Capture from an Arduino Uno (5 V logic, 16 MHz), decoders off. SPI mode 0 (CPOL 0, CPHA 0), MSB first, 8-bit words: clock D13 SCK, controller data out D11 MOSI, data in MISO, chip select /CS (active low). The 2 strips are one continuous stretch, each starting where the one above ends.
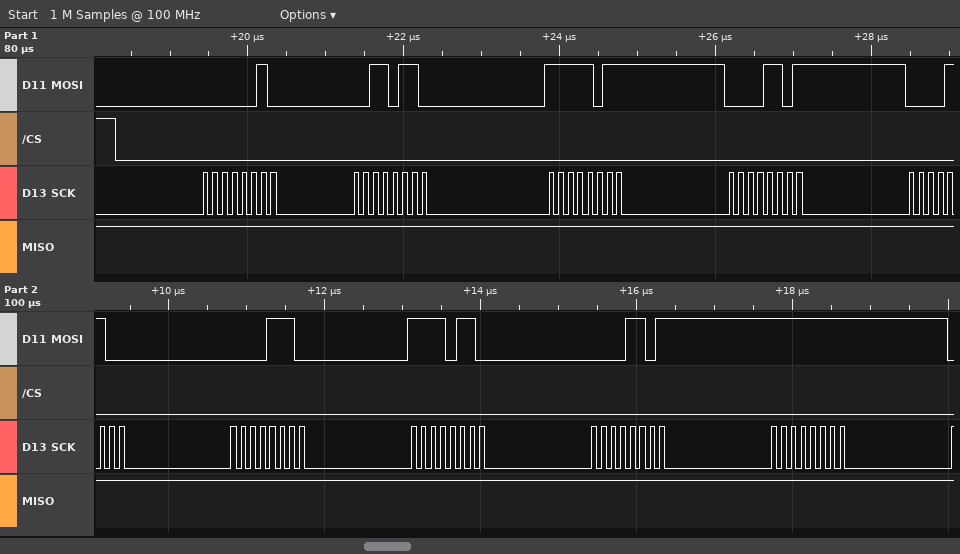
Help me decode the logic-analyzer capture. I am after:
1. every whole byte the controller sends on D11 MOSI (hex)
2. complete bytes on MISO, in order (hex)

0x02 0x36 0xFB 0x0D 0x0C 0x0E 0xF6 0x0D 0xFF
0xFF 0xFF 0xFF 0xFF 0xFF 0xFF 0xFF 0xFF 0xFF
